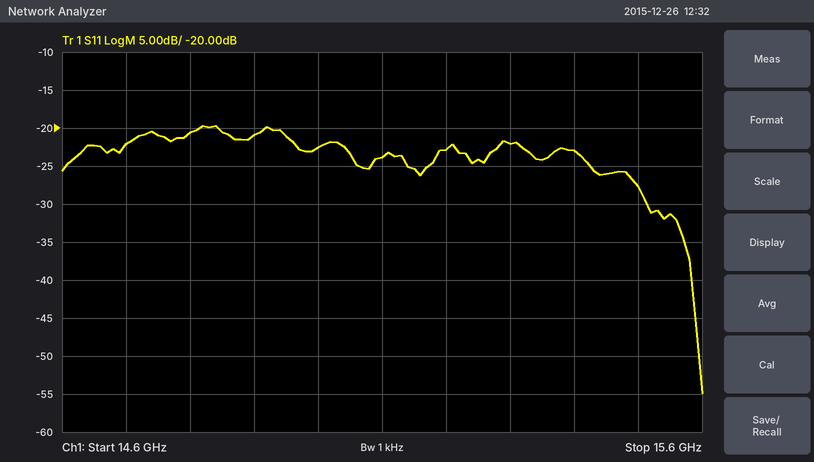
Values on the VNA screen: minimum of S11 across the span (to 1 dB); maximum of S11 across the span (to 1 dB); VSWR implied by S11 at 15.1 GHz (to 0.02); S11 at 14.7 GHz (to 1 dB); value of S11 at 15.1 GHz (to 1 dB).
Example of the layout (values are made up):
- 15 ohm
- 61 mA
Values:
- -55 dB
- -20 dB
- 1.14
- -22 dB
- -24 dB
